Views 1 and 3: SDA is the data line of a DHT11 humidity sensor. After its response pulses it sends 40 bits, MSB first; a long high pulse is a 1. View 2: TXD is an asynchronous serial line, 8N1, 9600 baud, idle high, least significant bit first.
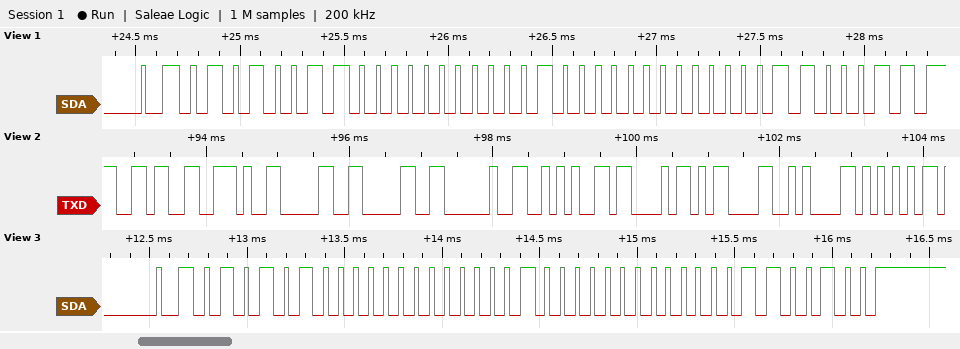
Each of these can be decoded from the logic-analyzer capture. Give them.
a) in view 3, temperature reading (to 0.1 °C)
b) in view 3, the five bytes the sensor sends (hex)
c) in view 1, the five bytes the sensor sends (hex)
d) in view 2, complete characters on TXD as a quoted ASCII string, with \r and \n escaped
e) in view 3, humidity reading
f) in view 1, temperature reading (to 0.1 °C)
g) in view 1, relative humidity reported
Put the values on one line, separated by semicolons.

16.0 °C; 54 00 10 00 64; 53 00 10 00 63; "6.00 *C\r\nU"; 84 %; 16.0 °C; 83 %
